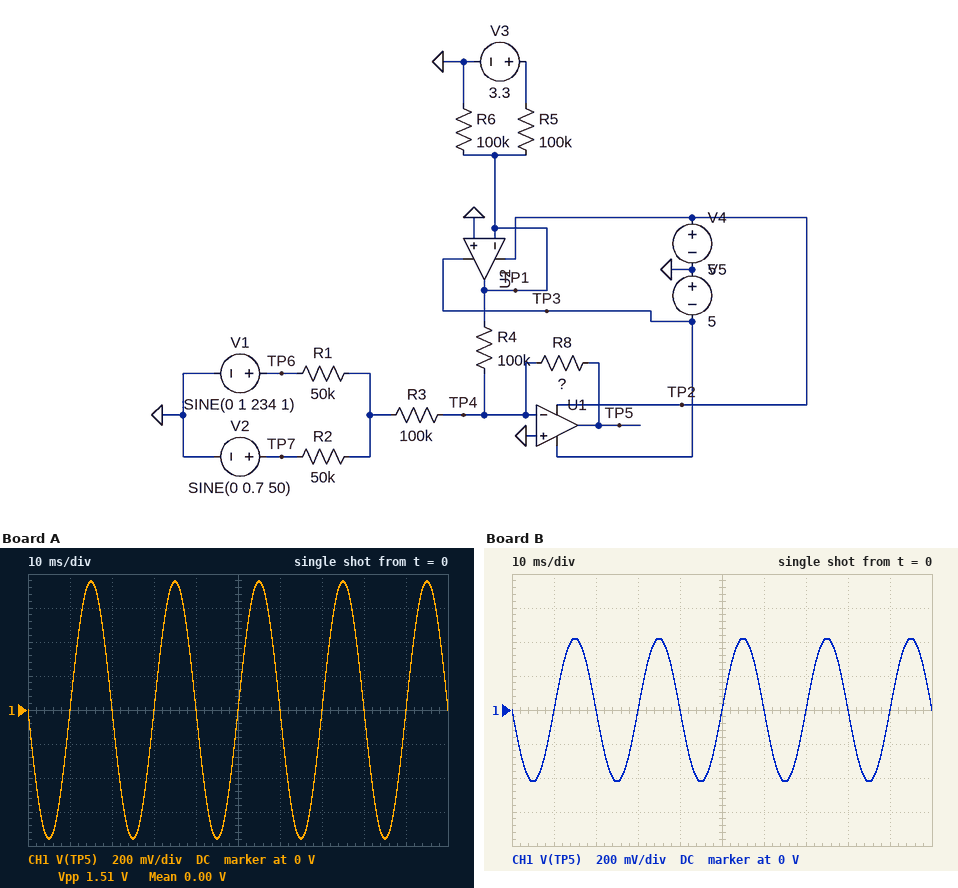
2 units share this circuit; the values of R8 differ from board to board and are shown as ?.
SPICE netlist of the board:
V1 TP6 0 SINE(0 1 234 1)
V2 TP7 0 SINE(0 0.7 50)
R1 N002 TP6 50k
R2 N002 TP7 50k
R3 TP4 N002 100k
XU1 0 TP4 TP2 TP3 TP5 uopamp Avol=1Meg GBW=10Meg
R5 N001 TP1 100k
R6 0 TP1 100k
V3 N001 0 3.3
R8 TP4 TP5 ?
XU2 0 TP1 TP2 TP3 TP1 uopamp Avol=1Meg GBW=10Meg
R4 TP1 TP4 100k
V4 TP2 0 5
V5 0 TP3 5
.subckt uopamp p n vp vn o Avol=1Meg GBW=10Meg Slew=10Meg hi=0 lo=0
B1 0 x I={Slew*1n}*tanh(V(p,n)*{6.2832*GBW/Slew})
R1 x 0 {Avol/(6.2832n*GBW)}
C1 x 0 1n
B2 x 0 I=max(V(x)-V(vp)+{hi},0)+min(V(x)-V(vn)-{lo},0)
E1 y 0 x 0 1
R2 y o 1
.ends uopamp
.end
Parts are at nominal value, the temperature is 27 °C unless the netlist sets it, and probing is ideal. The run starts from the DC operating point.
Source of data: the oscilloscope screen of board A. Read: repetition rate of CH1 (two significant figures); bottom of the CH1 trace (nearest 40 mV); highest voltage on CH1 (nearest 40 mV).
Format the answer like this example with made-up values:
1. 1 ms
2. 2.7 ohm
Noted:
1. 50 Hz
2. -760 mV
3. 760 mV
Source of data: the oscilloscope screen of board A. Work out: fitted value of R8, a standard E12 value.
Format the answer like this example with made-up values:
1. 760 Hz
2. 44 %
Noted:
1. 270 kΩ
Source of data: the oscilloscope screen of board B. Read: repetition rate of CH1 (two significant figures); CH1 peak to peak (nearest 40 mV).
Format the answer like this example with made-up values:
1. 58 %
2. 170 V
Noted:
1. 50 Hz
2. 840 mV
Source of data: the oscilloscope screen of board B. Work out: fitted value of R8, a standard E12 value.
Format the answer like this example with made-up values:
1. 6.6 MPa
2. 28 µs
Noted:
1. 150 kΩ
